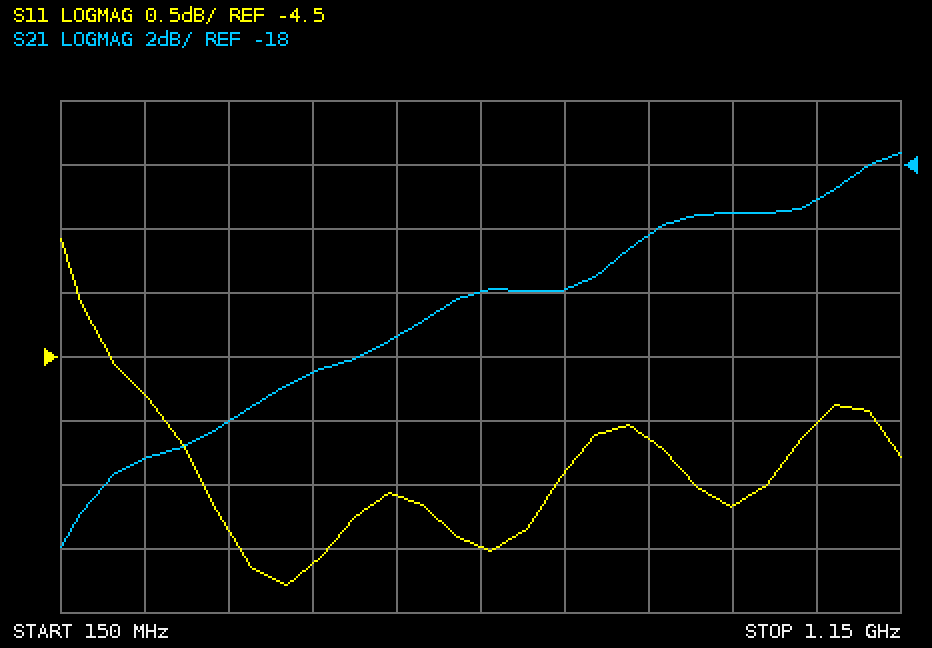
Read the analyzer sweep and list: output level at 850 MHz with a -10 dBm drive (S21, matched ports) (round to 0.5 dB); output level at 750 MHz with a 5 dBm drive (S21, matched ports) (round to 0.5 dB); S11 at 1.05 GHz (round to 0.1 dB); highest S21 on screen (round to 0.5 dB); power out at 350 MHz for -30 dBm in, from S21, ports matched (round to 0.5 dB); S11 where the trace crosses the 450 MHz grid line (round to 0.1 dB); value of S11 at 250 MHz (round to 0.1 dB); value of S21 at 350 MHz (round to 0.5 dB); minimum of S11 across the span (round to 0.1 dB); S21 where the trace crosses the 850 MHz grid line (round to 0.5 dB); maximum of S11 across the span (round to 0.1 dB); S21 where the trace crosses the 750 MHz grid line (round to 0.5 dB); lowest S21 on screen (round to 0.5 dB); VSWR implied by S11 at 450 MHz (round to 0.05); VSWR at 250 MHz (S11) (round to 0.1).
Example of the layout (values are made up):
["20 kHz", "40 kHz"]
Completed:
["-30.0 dBm", "-17.0 dBm", "-5.0 dB", "-17.5 dB", "-56.0 dBm", "-6.1 dB", "-4.8 dB", "-26.0 dB", "-6.3 dB", "-20.0 dB", "-3.6 dB", "-22.0 dB", "-30.0 dB", "2.95", "3.7"]
